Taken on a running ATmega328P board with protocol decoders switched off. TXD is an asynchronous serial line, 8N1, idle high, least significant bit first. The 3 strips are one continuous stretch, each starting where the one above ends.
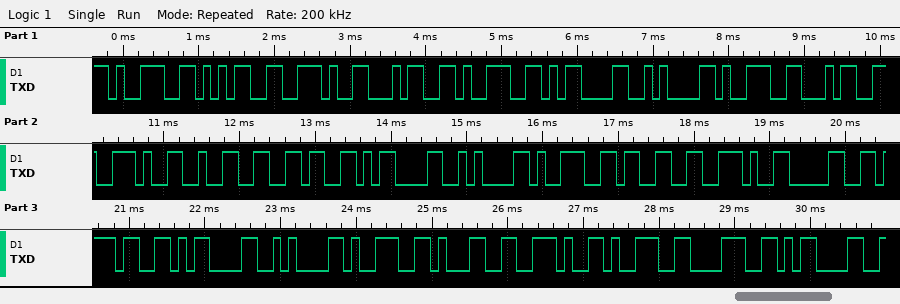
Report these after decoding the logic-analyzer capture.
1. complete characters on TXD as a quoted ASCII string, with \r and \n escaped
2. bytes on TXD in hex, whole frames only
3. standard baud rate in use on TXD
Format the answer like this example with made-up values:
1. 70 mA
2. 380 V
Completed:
1. "95.49\r\n94.26\r\n93.07\r\n91.98\r"
2. 39 35 2E 34 39 0D 0A 39 34 2E 32 36 0D 0A 39 33 2E 30 37 0D 0A 39 31 2E 39 38 0D
3. 9600 baud
